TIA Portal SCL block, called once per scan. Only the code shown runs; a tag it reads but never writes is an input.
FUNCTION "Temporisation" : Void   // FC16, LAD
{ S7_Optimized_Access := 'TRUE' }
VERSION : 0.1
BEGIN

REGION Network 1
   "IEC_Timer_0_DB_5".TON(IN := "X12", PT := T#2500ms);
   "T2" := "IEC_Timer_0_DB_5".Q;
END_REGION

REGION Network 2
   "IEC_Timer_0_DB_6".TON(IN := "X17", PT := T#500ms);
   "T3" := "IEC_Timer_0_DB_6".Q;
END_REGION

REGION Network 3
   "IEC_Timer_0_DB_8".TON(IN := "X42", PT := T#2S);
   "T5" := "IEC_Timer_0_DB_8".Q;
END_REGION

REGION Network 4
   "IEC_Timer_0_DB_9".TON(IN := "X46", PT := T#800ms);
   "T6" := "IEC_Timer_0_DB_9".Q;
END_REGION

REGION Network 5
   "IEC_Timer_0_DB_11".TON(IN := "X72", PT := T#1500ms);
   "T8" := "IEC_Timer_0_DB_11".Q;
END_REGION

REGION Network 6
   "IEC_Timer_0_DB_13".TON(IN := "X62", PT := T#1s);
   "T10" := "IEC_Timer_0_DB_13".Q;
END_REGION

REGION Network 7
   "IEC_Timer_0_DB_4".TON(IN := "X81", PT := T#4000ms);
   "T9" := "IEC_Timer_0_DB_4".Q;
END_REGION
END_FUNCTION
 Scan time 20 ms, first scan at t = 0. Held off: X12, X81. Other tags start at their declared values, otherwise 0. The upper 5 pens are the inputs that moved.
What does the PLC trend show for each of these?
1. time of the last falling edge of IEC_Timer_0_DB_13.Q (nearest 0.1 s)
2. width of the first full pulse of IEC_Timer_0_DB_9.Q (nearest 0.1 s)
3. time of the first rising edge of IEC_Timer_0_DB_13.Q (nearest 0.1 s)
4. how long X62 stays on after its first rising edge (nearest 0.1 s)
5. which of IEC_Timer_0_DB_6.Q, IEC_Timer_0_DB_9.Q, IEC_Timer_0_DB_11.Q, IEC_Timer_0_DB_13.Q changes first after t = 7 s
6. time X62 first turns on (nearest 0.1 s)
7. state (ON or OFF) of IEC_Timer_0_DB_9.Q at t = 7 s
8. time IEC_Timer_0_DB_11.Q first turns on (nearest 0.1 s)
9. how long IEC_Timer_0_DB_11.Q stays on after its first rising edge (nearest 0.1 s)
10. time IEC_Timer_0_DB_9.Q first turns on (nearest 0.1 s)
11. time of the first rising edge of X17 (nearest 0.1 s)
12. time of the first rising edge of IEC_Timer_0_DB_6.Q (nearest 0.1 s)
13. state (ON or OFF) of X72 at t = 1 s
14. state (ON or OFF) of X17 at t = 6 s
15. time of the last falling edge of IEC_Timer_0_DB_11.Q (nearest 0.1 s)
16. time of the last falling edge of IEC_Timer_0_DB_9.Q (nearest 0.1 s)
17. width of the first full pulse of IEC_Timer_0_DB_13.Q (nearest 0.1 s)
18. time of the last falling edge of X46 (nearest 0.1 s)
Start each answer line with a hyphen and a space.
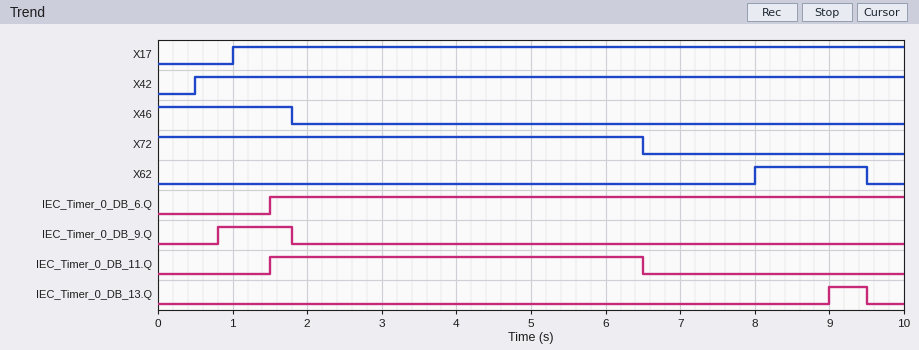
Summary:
- 9.5 s
- 1.0 s
- 9.0 s
- 1.5 s
- IEC_Timer_0_DB_13.Q
- 8.0 s
- OFF
- 1.5 s
- 5.0 s
- 0.8 s
- 1.0 s
- 1.5 s
- ON
- ON
- 6.5 s
- 1.8 s
- 0.5 s
- 1.8 s
